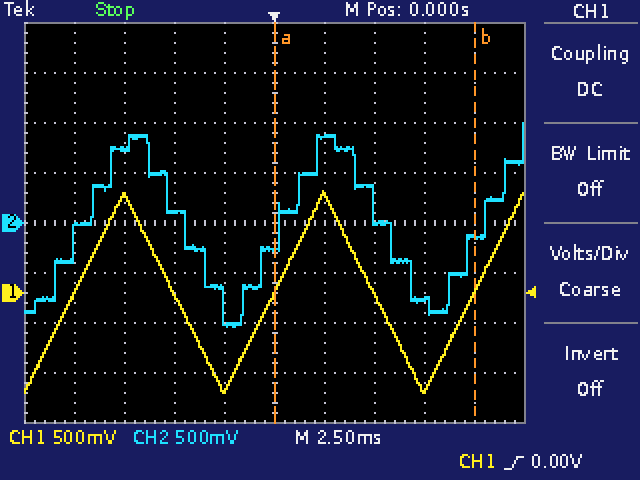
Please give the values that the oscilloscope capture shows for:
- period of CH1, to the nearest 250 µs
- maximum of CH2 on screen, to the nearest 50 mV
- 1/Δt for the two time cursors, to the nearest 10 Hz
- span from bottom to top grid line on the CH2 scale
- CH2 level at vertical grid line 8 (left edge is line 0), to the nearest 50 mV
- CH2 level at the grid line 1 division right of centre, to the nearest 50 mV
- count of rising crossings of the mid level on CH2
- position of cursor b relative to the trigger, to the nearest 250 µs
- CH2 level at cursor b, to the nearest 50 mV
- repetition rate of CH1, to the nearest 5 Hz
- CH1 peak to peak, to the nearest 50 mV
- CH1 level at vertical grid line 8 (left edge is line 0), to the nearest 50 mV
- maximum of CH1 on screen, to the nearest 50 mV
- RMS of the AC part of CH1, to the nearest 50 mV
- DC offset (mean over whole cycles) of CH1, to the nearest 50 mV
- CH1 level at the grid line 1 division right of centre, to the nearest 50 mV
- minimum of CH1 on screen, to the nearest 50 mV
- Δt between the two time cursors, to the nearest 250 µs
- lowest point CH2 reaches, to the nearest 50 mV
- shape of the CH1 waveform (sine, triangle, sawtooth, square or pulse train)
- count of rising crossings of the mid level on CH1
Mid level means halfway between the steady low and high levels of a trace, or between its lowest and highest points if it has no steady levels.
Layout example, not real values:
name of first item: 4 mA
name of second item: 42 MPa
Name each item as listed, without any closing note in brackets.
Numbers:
period of CH1, to the nearest 250 µs: 10.00 ms
maximum of CH2 on screen, to the nearest 50 mV: 1.00 V
1/Δt for the two time cursors, to the nearest 10 Hz: 100 Hz
span from bottom to top grid line on the CH2 scale: 4 V
CH2 level at vertical grid line 8 (left edge is line 0), to the nearest 50 mV: -750 mV
CH2 level at the grid line 1 division right of centre, to the nearest 50 mV: 850 mV
count of rising crossings of the mid level on CH2: 3
position of cursor b relative to the trigger, to the nearest 250 µs: +10.00 ms
CH2 level at cursor b, to the nearest 50 mV: -150 mV
repetition rate of CH1, to the nearest 5 Hz: 100 Hz
CH1 peak to peak, to the nearest 50 mV: 2.00 V
CH1 level at vertical grid line 8 (left edge is line 0), to the nearest 50 mV: -950 mV
maximum of CH1 on screen, to the nearest 50 mV: 1.00 V
RMS of the AC part of CH1, to the nearest 50 mV: 600 mV
DC offset (mean over whole cycles) of CH1, to the nearest 50 mV: 0 mV
CH1 level at the grid line 1 division right of centre, to the nearest 50 mV: 950 mV
minimum of CH1 on screen, to the nearest 50 mV: -1.00 V
Δt between the two time cursors, to the nearest 250 µs: 10.00 ms
lowest point CH2 reaches, to the nearest 50 mV: -1.05 V
shape of the CH1 waveform: triangle
count of rising crossings of the mid level on CH1: 3
